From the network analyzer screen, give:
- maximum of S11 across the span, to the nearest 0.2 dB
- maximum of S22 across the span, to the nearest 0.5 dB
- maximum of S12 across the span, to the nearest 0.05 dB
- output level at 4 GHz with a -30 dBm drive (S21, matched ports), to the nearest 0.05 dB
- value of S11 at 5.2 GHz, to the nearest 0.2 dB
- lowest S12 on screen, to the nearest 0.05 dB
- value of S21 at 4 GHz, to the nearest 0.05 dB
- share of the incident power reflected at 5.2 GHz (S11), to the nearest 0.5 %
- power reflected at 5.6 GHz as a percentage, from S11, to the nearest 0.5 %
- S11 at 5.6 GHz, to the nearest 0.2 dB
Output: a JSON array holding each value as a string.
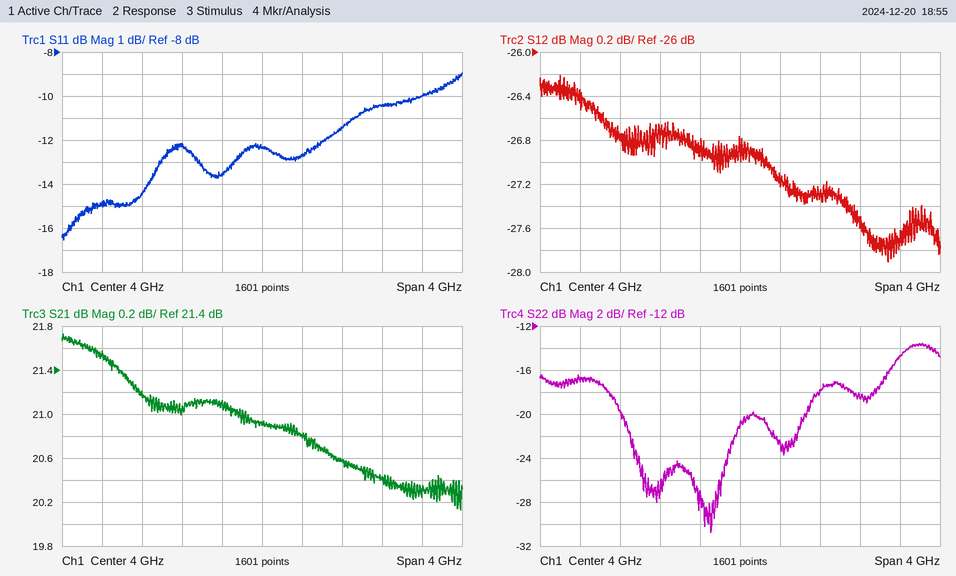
["-9.0 dB", "-13.5 dB", "-26.20 dB", "-9.10 dBm", "-10.4 dB", "-27.90 dB", "20.90 dB", "9.0 %", "10.0 %", "-10.0 dB"]
